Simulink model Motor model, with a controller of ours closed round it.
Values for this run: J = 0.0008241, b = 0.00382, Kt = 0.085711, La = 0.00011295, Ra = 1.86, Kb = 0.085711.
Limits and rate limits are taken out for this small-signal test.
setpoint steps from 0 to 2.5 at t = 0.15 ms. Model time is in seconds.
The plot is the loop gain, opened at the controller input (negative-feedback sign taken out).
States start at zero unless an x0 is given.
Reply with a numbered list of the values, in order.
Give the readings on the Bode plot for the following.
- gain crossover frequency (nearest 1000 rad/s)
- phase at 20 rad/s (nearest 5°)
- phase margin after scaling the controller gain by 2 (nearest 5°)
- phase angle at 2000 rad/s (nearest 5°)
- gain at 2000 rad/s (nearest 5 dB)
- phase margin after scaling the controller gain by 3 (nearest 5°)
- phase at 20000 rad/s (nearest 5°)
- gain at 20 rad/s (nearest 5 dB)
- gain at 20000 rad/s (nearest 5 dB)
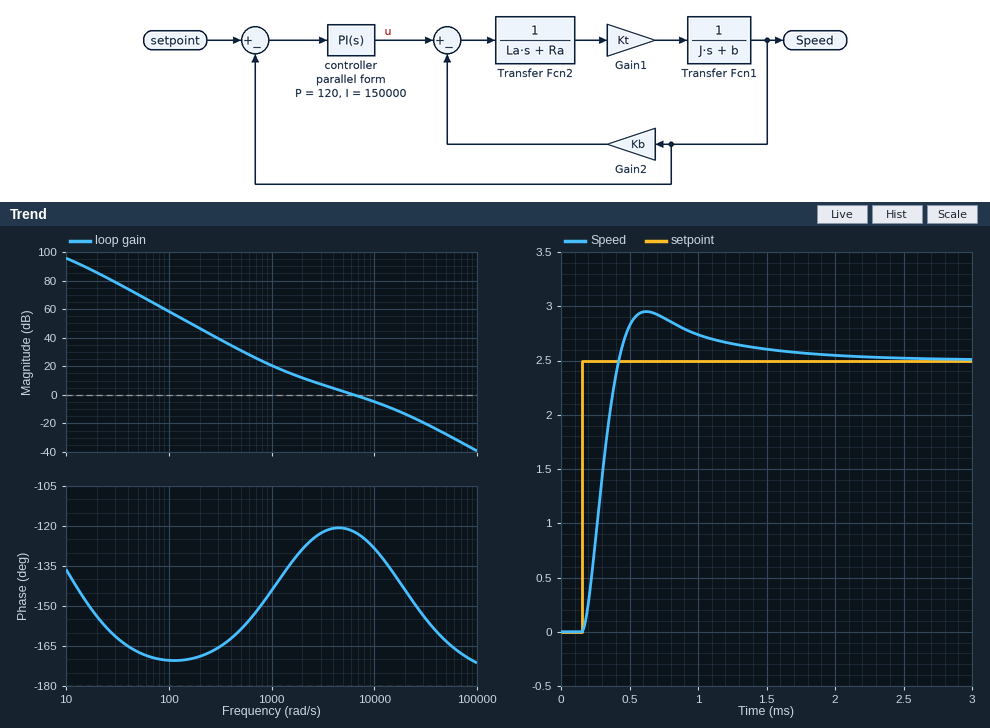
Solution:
1. 6000 rad/s
2. -155°
3. 50°
4. -130°
5. 10 dB
6. 45°
7. -145°
8. 85 dB
9. -15 dB
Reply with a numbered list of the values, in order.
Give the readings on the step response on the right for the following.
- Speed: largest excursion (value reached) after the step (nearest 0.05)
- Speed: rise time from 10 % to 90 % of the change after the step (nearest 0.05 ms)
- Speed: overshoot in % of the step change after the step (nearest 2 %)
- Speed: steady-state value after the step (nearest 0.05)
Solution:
1. 2.95
2. 0.20 ms
3. 18 %
4. 2.50
